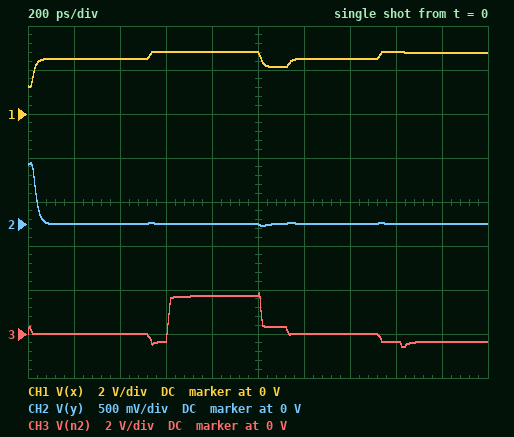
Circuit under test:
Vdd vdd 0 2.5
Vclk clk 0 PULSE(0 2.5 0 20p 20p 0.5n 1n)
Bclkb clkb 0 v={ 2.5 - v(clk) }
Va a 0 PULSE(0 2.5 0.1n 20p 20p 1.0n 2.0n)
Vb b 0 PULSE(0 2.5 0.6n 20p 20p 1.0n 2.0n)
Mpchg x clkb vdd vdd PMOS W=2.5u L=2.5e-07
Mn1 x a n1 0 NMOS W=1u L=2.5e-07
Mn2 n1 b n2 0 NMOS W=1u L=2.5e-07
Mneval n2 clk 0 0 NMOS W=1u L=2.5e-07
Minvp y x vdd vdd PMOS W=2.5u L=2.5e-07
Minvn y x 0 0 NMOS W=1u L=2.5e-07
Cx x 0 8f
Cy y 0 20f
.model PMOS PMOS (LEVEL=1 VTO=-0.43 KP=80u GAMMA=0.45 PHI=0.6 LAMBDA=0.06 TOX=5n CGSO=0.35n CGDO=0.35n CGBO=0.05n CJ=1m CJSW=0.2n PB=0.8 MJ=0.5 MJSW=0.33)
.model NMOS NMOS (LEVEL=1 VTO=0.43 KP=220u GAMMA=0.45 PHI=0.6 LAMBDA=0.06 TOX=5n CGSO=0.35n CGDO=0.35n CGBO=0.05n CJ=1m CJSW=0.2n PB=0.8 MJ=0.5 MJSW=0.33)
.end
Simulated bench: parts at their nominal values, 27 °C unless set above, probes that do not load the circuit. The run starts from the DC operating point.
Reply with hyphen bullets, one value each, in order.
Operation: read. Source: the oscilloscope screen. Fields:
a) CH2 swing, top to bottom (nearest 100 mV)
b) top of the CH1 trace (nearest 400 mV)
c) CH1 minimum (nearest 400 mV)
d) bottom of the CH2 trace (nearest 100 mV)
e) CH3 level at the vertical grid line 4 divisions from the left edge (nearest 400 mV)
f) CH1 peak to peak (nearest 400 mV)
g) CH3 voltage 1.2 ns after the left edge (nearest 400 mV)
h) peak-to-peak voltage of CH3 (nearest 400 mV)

- 700 mV
- 2.8 V
- 1.2 V
- 0 V
- 1.6 V
- 1.6 V
- 0 V
- 2.4 V
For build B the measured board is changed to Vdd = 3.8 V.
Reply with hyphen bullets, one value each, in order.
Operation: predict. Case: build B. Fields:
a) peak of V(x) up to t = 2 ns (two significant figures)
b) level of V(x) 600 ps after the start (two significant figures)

- 4.0 V
- 3.8 V
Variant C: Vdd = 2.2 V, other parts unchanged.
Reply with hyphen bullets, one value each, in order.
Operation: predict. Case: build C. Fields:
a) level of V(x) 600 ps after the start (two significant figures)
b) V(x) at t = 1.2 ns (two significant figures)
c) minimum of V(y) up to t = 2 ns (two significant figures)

- 2.5 V
- 2.2 V
- -25 mV
